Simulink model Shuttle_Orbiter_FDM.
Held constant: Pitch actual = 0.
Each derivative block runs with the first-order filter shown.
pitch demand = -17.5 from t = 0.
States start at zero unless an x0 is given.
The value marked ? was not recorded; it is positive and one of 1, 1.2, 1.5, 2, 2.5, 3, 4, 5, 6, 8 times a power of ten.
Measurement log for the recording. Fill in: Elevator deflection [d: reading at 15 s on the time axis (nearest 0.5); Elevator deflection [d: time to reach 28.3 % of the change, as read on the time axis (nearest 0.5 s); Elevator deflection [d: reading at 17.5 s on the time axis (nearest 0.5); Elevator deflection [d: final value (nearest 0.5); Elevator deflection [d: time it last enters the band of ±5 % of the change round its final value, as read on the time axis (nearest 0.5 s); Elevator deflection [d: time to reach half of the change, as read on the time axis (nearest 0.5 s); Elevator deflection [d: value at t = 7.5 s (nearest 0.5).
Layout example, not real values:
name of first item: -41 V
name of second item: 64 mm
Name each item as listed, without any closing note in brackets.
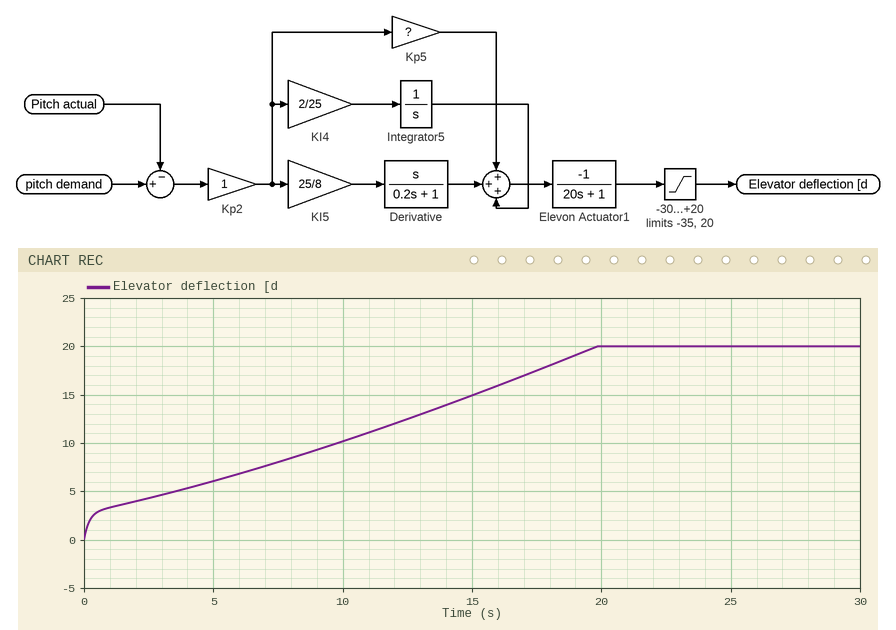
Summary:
Elevator deflection [d: reading at 15 s on the time axis: 15.0
Elevator deflection [d: time to reach 28.3 % of the change, as read on the time axis: 4.5 s
Elevator deflection [d: reading at 17.5 s on the time axis: 17.5
Elevator deflection [d: final value: 20.0
Elevator deflection [d: time it last enters the band of ±5 % of the change round its final value, as read on the time axis: 19.0 s
Elevator deflection [d: time to reach half of the change, as read on the time axis: 10.0 s
Elevator deflection [d: value at t = 7.5 s: 8.0
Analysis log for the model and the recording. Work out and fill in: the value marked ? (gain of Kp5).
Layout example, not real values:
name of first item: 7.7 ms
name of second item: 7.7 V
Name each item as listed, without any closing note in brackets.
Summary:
the value marked ?: 0.8
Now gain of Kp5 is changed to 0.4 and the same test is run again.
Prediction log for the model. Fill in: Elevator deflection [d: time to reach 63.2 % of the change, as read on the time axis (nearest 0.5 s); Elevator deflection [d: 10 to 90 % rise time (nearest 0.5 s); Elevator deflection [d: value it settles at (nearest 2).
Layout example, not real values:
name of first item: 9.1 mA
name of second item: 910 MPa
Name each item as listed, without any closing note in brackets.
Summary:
Elevator deflection [d: time to reach 63.2 % of the change, as read on the time axis: 16.5 s
Elevator deflection [d: 10 to 90 % rise time: 22.0 s
Elevator deflection [d: value it settles at: 20
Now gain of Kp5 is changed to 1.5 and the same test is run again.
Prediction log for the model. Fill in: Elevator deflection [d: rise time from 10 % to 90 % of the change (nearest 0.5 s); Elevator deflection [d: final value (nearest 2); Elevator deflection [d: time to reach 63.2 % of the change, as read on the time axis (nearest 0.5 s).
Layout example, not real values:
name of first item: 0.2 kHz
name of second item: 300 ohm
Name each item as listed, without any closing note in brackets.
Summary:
Elevator deflection [d: rise time from 10 % to 90 % of the change: 12.0 s
Elevator deflection [d: final value: 20
Elevator deflection [d: time to reach 63.2 % of the change, as read on the time axis: 8.0 s
